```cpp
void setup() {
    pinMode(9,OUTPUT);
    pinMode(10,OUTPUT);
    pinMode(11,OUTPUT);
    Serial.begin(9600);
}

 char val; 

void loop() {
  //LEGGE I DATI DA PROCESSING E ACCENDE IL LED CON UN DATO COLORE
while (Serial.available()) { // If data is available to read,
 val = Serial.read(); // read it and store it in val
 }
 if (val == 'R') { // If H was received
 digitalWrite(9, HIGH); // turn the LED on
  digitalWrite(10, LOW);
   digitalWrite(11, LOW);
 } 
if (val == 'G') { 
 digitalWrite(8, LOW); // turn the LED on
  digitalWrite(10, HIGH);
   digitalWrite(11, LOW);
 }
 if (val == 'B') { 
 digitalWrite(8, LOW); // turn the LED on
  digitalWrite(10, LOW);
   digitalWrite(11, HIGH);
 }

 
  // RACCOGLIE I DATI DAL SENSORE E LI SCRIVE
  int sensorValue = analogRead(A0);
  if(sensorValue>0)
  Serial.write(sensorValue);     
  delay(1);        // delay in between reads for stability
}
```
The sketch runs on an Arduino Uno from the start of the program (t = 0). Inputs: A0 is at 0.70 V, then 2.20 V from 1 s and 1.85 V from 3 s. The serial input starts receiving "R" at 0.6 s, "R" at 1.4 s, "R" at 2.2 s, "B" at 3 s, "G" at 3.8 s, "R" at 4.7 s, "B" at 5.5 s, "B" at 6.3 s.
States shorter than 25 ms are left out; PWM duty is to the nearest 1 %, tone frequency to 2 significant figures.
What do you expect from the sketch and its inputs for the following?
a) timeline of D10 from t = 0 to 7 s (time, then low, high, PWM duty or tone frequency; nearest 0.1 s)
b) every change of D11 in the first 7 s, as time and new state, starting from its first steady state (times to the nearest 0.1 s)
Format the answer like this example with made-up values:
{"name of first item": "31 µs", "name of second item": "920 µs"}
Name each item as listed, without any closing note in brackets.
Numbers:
{"timeline of D10 from t = 0 to 7 s": "0 s low; 3.8 s high; 4.7 s low", "every change of D11 in the first 7 s, as time and new state, starting from its first steady state": "0 s low; 3 s high; 3.8 s low; 5.5 s high"}
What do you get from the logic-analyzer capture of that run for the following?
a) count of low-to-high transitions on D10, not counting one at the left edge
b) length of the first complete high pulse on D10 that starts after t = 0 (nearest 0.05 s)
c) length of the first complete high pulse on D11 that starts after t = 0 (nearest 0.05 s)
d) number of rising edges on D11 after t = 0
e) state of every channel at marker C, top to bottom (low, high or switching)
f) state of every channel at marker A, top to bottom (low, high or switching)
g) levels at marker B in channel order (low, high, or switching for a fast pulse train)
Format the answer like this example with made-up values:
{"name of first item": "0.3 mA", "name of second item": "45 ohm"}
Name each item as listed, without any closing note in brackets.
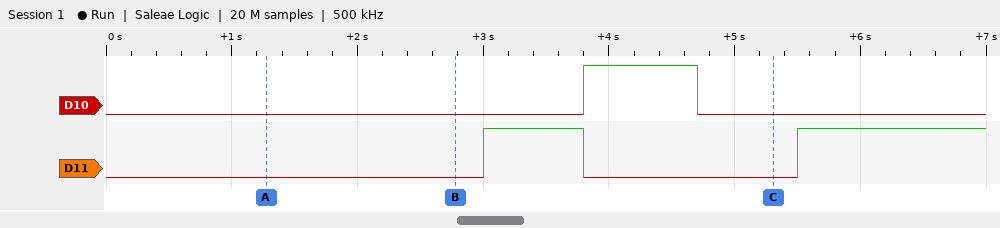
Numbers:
{"count of low-to-high transitions on D10, not counting one at the left edge": "1", "length of the first complete high pulse on D10 that starts after t = 0": "0.90 s", "length of the first complete high pulse on D11 that starts after t = 0": "0.80 s", "number of rising edges on D11 after t = 0": "2", "state of every channel at marker C, top to bottom": "D10 low, D11 low", "state of every channel at marker A, top to bottom": "D10 low, D11 low", "levels at marker B in channel order": "D10 low, D11 low"}
